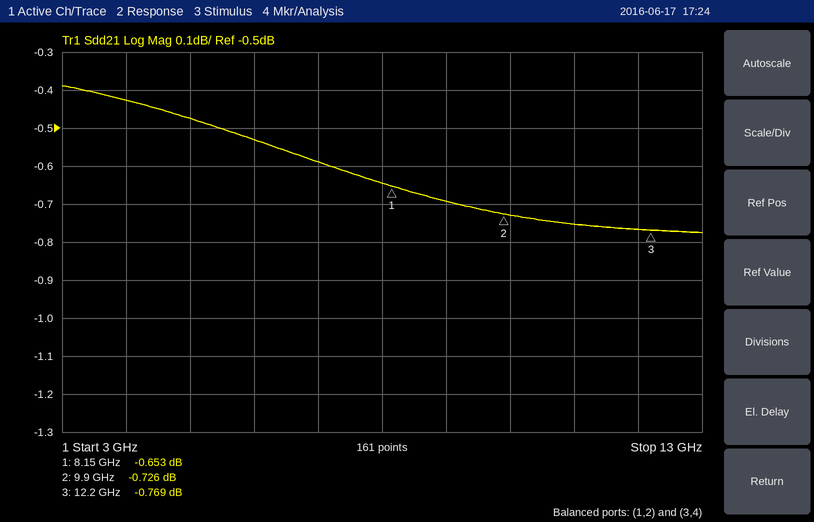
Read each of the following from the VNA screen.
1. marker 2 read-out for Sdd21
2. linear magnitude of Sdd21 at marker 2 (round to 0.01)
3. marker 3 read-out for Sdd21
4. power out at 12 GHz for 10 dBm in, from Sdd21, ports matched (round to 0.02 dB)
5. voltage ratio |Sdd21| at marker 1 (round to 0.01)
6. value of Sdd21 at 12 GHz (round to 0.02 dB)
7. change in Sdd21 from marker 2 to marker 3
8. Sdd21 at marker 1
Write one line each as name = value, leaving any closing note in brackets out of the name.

marker 2 read-out for Sdd21 = -0.726 dB
linear magnitude of Sdd21 at marker 2 = 0.92
marker 3 read-out for Sdd21 = -0.769 dB
power out at 12 GHz for 10 dBm in, from Sdd21, ports matched = 9.24 dBm
voltage ratio |Sdd21| at marker 1 = 0.93
value of Sdd21 at 12 GHz = -0.76 dB
change in Sdd21 from marker 2 to marker 3 = -0.043 dB
Sdd21 at marker 1 = -0.653 dB
